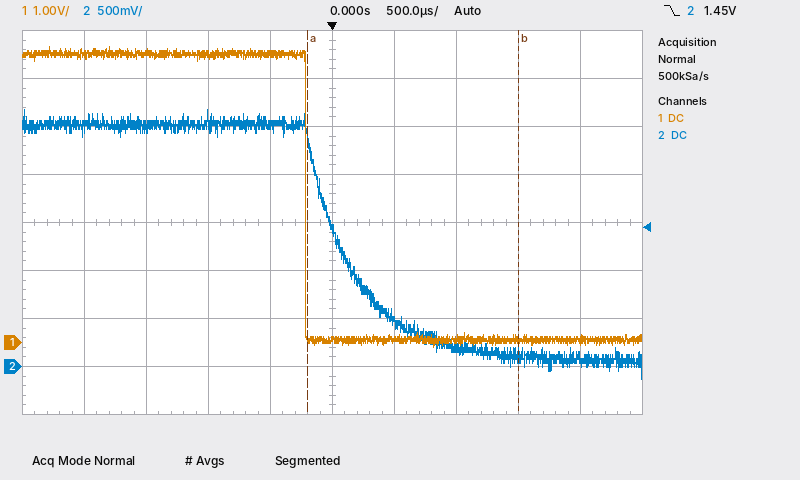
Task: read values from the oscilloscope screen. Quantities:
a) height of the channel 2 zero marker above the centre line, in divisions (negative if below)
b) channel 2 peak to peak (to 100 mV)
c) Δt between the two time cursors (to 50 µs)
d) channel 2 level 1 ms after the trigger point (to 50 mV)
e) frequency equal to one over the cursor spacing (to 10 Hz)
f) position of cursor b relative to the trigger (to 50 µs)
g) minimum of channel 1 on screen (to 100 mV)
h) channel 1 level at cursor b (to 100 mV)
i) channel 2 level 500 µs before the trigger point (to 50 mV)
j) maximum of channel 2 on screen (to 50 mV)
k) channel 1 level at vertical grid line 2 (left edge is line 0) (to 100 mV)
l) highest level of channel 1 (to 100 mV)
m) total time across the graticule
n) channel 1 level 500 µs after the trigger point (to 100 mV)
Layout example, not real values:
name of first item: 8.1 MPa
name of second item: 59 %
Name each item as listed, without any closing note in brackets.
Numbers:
height of the channel 2 zero marker above the centre line, in divisions: -3.0 div
channel 2 peak to peak: 2.80 V
Δt between the two time cursors: 1.70 ms
channel 2 level 1 ms after the trigger point: 200 mV
frequency equal to one over the cursor spacing: 590 Hz
position of cursor b relative to the trigger: +1.50 ms
minimum of channel 1 on screen: -100 mV
channel 1 level at cursor b: 100 mV
channel 2 level 500 µs before the trigger point: 2.50 V
maximum of channel 2 on screen: 2.70 V
channel 1 level at vertical grid line 2 (left edge is line 0): 6.0 V
highest level of channel 1: 6.2 V
total time across the graticule: 5 ms
channel 1 level 500 µs after the trigger point: 100 mV
